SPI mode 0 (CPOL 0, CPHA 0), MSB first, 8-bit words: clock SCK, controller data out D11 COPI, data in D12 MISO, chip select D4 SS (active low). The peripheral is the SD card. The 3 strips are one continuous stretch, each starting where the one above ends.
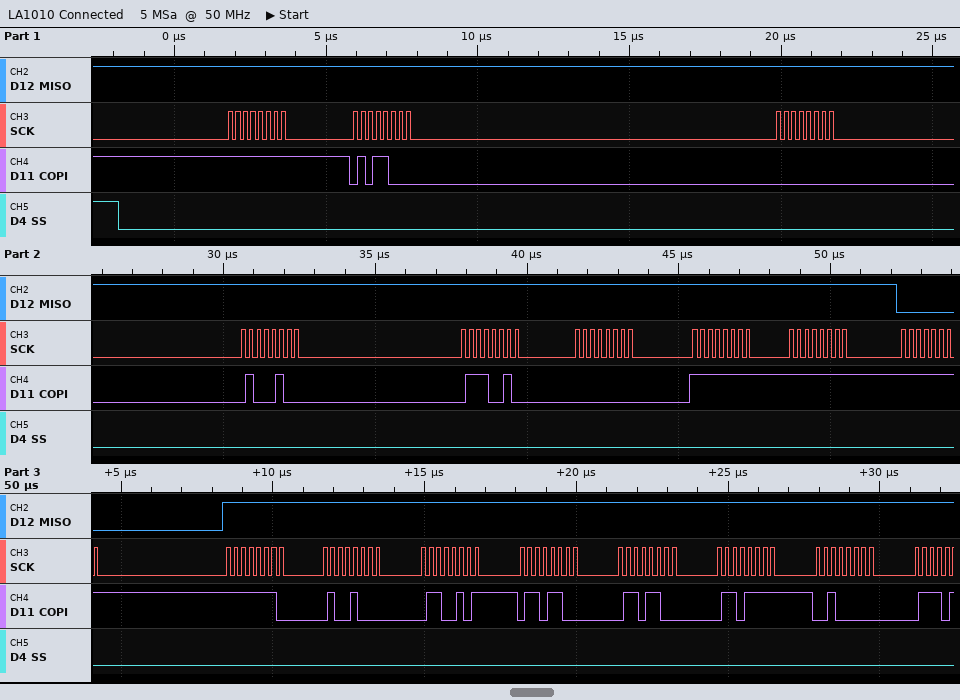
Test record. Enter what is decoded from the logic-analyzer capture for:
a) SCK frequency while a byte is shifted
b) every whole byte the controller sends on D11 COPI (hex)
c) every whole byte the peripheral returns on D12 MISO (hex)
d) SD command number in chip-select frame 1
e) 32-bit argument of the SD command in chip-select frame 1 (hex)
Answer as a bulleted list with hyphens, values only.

- 4 MHz
- FF 58 00 44 72 00 FF FF FF FE 48 65 6C 6C 6F 20
- FF FF FF FF FF FF FF FF 00 FF FF FF FF FF FF FF
- CMD24
- 0x00447200
